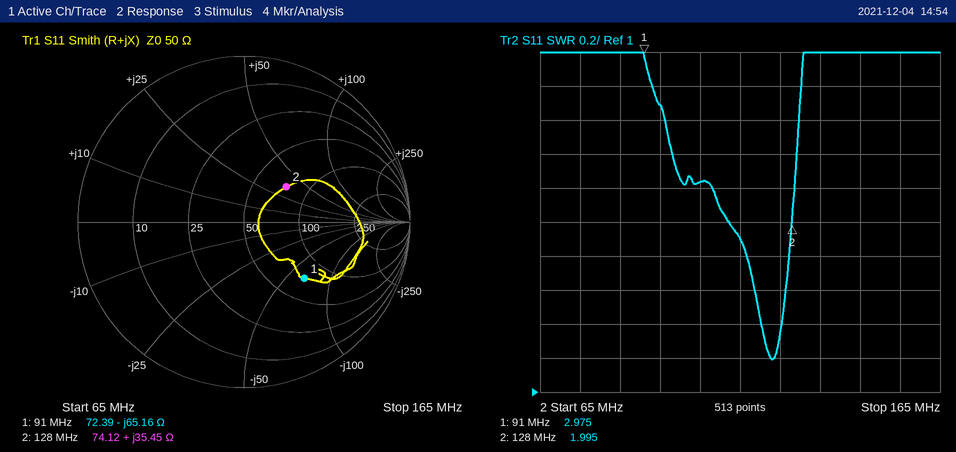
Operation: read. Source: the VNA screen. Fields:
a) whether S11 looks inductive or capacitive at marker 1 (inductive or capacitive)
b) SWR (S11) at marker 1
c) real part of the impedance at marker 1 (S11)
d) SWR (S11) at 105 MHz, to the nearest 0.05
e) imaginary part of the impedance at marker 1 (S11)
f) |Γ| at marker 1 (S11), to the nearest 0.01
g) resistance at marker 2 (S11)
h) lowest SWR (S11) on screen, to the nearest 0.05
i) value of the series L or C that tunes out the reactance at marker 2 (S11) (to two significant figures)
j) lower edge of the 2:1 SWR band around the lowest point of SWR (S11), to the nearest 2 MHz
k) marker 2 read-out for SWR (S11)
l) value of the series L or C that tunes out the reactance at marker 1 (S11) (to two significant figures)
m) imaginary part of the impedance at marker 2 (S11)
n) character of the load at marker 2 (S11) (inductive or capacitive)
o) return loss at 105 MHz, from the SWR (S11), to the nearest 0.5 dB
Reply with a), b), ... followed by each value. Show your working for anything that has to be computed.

a) capacitive
b) 2.975
c) 72.39 Ω
d) 2.25
e) -65.16 Ω
f) 0.50
g) 74.12 Ω
h) 1.20
i) C = 1/(2π × 128 MHz × 35.45 Ω) ≈ 35 pF
j) 112 MHz
k) 1.995
l) L = 65.16 Ω/(2π × 91 MHz) ≈ 114 nH, so 110 nH to two significant figures
m) +35.45 Ω
n) inductive
o) −20 log10((2.25 − 1)/(2.25 + 1)) ≈ 8.30 dB, so 8.5 dB to the nearest 0.5 dB
